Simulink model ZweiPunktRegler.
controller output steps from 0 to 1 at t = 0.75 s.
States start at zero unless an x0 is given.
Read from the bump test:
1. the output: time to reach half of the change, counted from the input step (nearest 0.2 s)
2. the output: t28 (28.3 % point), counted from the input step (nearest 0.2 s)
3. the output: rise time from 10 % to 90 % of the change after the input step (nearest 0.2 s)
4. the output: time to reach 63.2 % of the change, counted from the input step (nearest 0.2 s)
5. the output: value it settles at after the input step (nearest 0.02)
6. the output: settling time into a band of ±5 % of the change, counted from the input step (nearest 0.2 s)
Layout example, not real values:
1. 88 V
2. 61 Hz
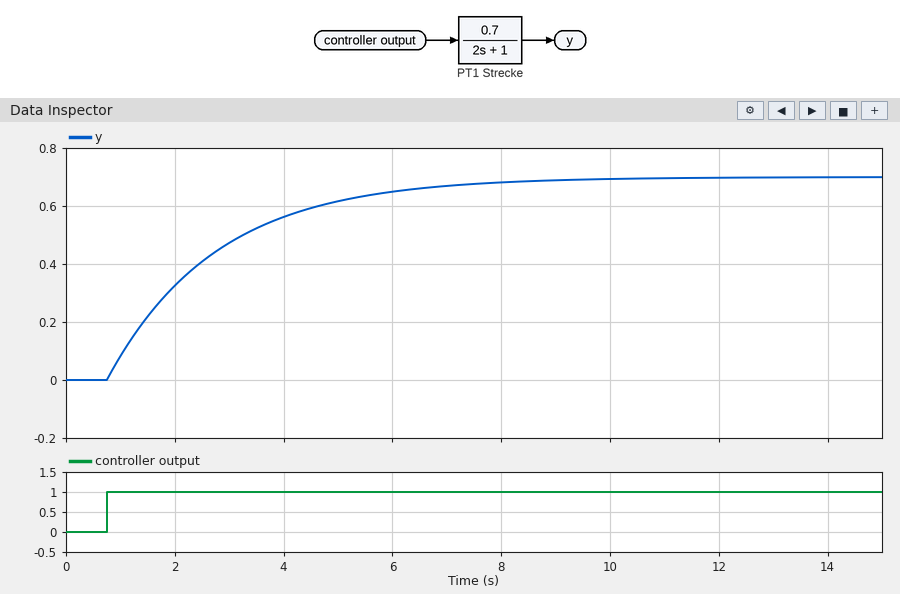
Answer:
1. 1.4 s
2. 0.6 s
3. 4.4 s
4. 2.0 s
5. 0.70
6. 6.0 s
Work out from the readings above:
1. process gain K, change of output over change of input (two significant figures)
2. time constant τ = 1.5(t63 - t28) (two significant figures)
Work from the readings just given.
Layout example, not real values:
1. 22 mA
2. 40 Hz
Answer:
1. 0.70
2. 2.1 s
